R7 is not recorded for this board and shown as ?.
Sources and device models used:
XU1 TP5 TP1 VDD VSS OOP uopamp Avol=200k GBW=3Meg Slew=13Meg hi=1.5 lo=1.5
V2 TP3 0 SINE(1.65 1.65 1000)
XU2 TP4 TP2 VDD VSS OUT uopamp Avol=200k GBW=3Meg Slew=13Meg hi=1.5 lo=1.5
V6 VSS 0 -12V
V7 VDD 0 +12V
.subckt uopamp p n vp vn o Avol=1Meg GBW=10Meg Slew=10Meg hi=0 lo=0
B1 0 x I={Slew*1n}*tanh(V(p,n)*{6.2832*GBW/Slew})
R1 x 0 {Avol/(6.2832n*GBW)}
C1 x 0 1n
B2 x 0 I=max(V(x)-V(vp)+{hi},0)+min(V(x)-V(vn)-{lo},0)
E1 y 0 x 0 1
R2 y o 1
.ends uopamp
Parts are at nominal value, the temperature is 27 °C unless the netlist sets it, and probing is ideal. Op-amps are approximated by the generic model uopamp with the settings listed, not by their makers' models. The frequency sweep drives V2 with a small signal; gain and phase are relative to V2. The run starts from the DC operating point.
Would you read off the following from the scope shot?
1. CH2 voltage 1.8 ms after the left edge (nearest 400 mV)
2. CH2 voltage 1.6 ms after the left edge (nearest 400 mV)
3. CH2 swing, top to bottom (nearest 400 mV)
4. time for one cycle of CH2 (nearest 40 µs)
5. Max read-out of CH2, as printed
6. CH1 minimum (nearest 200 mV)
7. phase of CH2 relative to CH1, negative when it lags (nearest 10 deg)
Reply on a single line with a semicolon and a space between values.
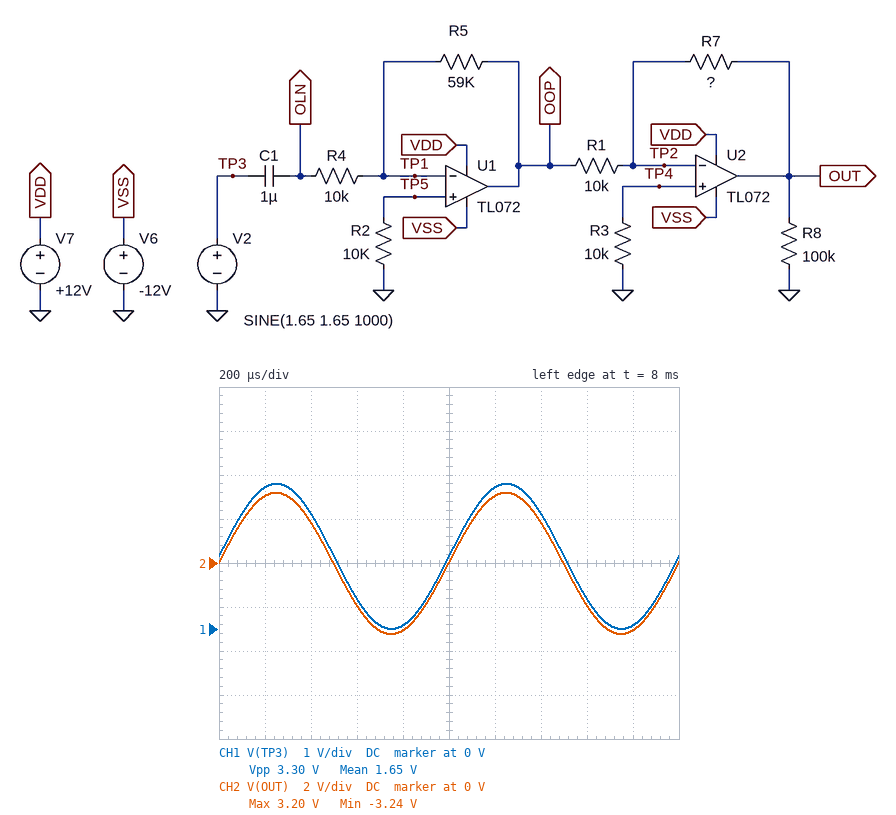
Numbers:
-3.2 V; -2.0 V; 6.4 V; 1.00 ms; 3.20 V; 0 V; 0 deg
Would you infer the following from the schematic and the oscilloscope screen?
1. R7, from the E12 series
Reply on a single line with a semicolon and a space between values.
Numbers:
3.3 kΩ
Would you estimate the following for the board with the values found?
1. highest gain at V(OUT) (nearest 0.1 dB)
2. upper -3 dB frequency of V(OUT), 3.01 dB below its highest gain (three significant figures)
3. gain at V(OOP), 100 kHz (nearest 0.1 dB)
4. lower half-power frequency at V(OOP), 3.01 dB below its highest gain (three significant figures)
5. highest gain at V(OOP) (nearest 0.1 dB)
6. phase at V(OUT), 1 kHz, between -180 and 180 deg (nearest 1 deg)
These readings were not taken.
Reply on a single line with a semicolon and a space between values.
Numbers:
5.8 dB; 420 kHz; 15.2 dB; 15.9 Hz; 15.4 dB; 1 deg
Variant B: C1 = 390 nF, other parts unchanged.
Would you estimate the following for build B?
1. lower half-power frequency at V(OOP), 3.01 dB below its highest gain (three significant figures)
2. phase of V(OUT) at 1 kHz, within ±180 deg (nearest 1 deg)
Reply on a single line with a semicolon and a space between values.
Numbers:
40.8 Hz; 2 deg
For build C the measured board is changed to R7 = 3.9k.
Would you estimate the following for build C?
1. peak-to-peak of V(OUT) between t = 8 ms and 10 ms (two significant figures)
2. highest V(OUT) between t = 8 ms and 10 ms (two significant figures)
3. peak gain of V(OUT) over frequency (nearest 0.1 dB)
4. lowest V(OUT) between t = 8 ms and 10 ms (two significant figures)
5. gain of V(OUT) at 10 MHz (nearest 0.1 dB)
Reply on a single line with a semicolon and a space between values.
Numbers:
7.6 V; 3.8 V; 7.2 dB; -3.8 V; -33.5 dB
